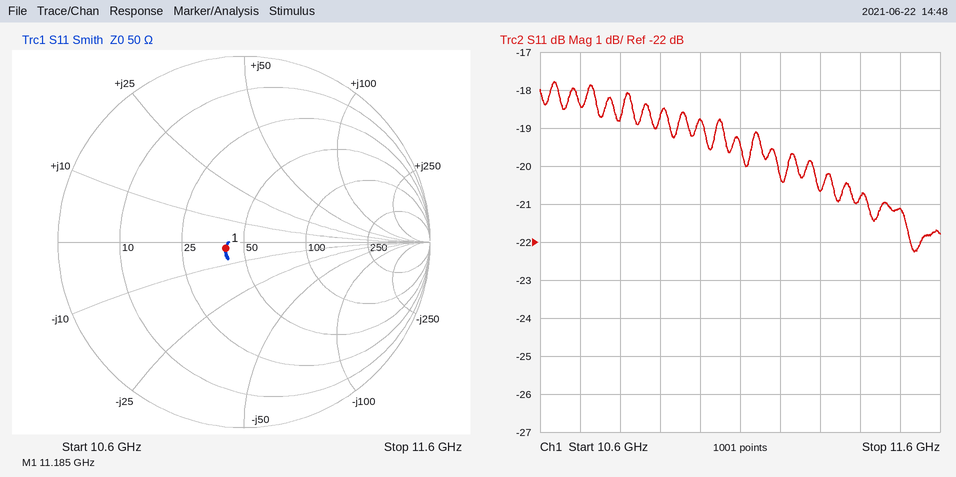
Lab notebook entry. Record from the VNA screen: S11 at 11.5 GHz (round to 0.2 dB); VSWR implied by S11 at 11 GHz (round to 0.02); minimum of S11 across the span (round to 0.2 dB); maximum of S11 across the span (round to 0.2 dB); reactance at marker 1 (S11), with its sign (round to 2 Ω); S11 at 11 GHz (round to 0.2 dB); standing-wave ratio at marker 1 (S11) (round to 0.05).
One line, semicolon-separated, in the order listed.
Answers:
-21.2 dB; 1.26; -22.2 dB; -17.8 dB; -2 Ω; -18.8 dB; 1.25
